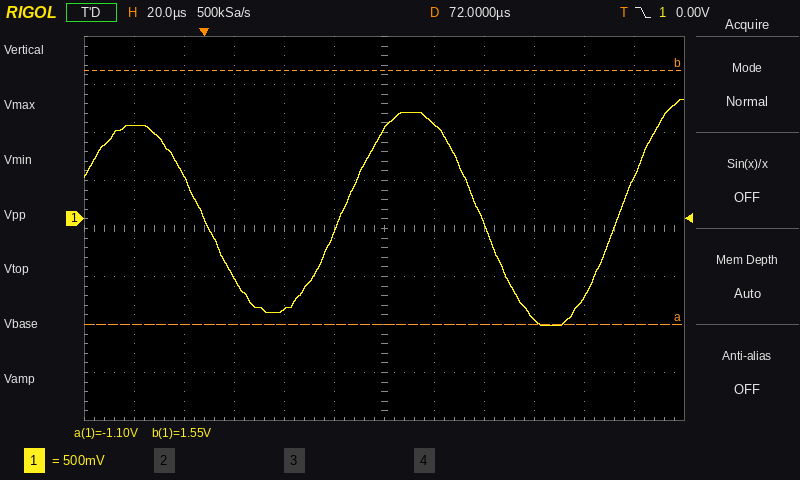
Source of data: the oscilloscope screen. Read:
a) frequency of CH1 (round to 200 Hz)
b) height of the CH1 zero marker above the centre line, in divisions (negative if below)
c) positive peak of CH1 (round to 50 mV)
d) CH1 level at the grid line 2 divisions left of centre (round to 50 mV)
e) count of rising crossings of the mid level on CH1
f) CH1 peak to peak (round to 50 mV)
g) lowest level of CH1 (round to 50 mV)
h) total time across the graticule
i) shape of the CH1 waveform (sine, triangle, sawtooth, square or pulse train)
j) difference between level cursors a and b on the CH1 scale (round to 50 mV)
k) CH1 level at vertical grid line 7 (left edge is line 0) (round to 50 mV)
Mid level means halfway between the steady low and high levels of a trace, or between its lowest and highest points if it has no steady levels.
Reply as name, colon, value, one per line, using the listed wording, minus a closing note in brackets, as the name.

frequency of CH1: 9.0 kHz
height of the CH1 zero marker above the centre line, in divisions: +0.2 div
positive peak of CH1: 1.25 V
CH1 level at the grid line 2 divisions left of centre: -950 mV
count of rising crossings of the mid level on CH1: 2
CH1 peak to peak: 2.35 V
lowest level of CH1: -1.10 V
total time across the graticule: 240 µs
shape of the CH1 waveform: sine
difference between level cursors a and b on the CH1 scale: 2.65 V
CH1 level at vertical grid line 7 (left edge is line 0): 1.00 V
